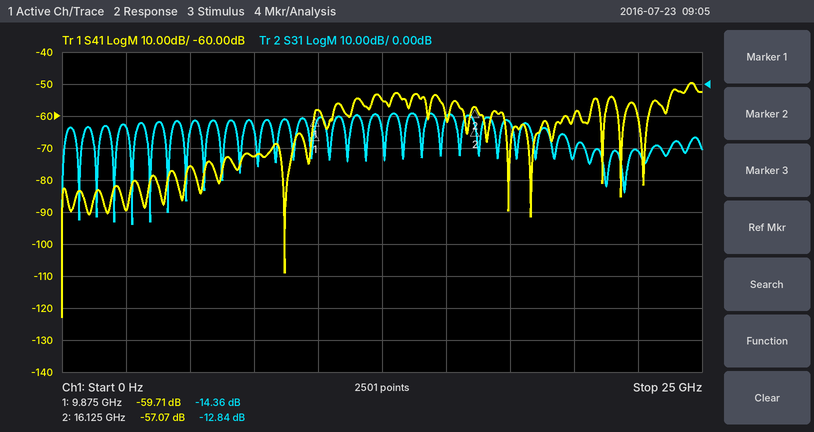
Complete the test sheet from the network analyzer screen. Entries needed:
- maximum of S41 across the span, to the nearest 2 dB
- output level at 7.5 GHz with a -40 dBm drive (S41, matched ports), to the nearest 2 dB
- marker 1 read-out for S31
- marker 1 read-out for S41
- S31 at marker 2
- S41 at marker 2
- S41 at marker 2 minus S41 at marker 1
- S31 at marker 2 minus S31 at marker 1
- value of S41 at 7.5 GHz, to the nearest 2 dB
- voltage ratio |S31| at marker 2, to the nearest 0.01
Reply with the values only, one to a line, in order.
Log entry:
-50 dB
-112 dBm
-14.36 dB
-59.71 dB
-12.84 dB
-57.07 dB
2.64 dB
1.52 dB
-72 dB
0.23
